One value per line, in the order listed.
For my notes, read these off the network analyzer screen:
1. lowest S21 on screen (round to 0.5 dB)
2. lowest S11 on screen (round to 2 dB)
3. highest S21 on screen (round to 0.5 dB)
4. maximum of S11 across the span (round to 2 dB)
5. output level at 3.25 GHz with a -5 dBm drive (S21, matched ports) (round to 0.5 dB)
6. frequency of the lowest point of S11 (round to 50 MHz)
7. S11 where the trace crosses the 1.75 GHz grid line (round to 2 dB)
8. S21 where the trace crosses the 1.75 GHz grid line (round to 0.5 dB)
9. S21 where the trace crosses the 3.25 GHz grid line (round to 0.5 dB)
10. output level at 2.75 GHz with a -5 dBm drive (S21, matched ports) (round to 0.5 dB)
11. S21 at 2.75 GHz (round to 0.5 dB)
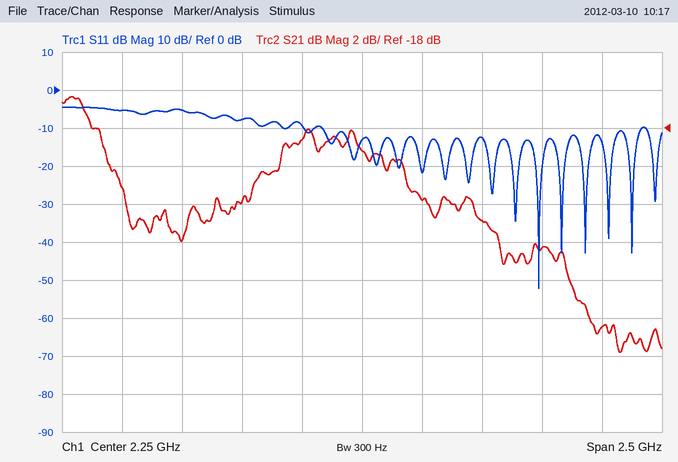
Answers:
-30.0 dB
-52 dB
-16.5 dB
-4 dB
-33.5 dBm
3.00 GHz
-8 dB
-22.0 dB
-28.5 dB
-28.0 dBm
-23.0 dB
